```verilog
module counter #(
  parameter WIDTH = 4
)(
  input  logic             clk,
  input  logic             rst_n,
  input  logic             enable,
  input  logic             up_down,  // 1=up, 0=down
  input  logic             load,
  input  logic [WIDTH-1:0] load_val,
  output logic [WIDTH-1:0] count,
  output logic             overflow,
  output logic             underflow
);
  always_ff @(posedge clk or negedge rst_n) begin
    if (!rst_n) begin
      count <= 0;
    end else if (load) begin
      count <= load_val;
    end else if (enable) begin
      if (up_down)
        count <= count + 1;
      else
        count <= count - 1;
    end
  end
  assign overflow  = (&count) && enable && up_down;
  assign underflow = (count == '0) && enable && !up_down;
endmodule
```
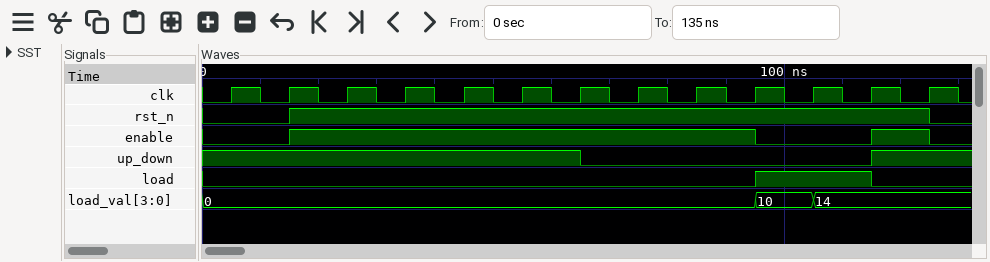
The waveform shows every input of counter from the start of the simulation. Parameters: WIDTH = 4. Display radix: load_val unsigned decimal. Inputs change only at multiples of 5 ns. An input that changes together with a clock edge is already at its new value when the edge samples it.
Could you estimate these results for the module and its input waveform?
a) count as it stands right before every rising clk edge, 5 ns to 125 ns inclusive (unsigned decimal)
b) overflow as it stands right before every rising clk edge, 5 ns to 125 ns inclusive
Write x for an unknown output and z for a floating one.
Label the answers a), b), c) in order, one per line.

a) 0, 0, 1, 2, 3, 4, 5, 4, 3, 2, 10, 14, 15
b) 0 0 0 0 0 0 0 0 0 0 0 0 1
